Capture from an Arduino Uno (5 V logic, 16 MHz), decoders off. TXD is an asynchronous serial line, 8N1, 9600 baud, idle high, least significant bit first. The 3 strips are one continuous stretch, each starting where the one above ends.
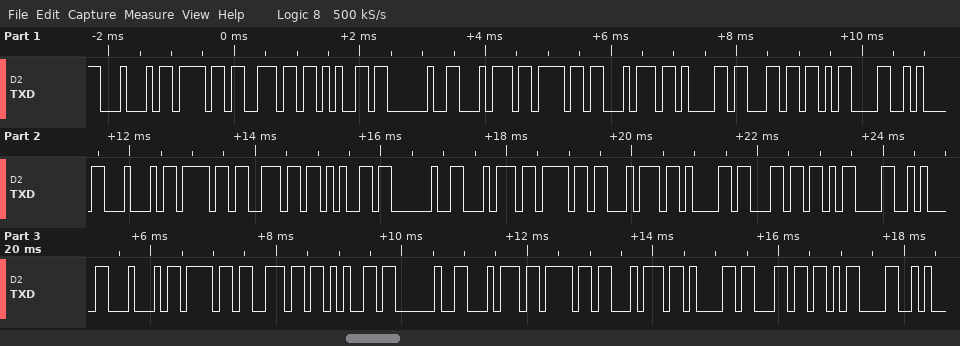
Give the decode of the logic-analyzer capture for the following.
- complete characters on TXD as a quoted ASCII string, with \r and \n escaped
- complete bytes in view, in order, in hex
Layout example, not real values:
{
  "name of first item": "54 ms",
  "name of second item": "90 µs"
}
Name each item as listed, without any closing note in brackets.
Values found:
{
  "complete characters on TXD as a quoted ASCII string, with \\r and \\n escaped": "\"Done total\\r\\nDone total\\r\\nDone total\\r\"",
  "complete bytes in view, in order, in hex": "44 6F 6E 65 20 74 6F 74 61 6C 0D 0A 44 6F 6E 65 20 74 6F 74 61 6C 0D 0A 44 6F 6E 65 20 74 6F 74 61 6C 0D"
}
